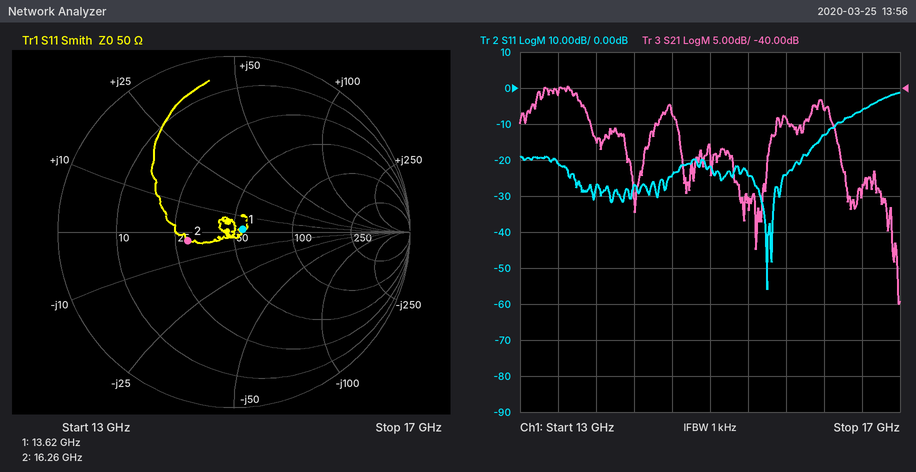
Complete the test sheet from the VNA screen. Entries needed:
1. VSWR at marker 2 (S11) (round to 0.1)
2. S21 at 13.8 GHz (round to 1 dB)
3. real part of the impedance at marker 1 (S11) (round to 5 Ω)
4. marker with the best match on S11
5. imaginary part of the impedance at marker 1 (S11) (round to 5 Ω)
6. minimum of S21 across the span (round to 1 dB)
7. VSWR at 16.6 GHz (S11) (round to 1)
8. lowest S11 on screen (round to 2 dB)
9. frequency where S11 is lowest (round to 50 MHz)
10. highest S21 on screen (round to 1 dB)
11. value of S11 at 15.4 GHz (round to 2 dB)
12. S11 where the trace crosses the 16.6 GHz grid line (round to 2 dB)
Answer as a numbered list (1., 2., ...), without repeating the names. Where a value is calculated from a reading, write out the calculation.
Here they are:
1. 1.7
2. -47 dB
3. 55 Ω
4. marker 1
5. 0 Ω
6. -70 dB
7. |Γ| = 10^(-6/20) = 0.5012; VSWR = (1 + 0.5012)/(1 − 0.5012) ≈ 3
8. -56 dB
9. 15.60 GHz
10. -40 dB
11. -24 dB
12. -6 dB
